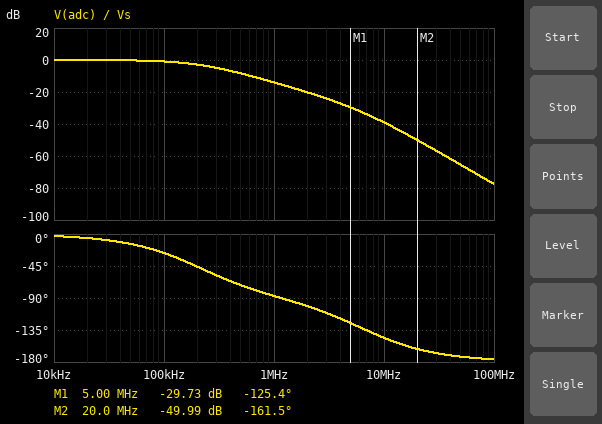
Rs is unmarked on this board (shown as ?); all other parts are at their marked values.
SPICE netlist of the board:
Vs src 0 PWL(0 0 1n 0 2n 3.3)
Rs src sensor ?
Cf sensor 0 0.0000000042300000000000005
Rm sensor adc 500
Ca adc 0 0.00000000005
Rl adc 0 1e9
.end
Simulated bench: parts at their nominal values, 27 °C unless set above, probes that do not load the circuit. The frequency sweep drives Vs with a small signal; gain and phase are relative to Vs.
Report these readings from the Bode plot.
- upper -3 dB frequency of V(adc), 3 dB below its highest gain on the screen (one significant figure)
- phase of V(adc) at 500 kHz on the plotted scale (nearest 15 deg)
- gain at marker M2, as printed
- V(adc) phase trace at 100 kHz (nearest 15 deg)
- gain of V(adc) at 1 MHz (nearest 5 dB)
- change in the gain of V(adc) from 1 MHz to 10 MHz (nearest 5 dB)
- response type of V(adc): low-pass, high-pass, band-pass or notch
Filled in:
200 kHz
-75 deg
-49.99 dB
-30 deg
-15 dB
-25 dB
low-pass
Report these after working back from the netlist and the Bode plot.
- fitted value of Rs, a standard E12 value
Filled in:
180 Ω
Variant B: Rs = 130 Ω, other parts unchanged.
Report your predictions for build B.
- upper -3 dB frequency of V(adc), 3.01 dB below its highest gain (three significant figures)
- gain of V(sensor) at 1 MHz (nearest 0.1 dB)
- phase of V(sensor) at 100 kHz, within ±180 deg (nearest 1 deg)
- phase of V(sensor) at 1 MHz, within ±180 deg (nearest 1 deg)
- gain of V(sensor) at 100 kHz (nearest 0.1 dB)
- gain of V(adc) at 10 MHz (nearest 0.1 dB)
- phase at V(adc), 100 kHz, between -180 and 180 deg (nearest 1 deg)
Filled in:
285 kHz
-11.2 dB
-19 deg
-74 deg
-0.5 dB
-36.2 dB
-20 deg
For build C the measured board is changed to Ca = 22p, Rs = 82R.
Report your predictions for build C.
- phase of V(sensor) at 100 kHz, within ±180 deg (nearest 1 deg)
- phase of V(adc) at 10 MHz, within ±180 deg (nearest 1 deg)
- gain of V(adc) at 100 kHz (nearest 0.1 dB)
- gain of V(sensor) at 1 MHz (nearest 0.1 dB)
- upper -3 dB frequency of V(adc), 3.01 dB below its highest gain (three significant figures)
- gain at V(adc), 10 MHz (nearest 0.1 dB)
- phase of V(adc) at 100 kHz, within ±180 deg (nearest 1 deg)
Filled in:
-12 deg
-122 deg
-0.2 dB
-7.6 dB
456 kHz
-28.5 dB
-13 deg
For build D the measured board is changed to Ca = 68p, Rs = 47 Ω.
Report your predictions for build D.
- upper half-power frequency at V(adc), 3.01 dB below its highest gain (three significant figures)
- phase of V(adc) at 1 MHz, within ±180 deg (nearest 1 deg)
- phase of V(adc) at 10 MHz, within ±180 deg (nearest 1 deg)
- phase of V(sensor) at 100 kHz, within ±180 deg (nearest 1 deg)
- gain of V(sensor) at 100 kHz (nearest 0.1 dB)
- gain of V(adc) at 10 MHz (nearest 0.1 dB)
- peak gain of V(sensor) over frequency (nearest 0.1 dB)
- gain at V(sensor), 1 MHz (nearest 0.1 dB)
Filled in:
765 kHz
-64 deg
-150 deg
-7 deg
-0.1 dB
-29.4 dB
0 dB
-4.2 dB
